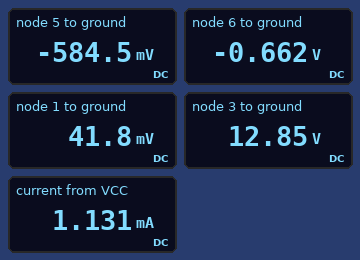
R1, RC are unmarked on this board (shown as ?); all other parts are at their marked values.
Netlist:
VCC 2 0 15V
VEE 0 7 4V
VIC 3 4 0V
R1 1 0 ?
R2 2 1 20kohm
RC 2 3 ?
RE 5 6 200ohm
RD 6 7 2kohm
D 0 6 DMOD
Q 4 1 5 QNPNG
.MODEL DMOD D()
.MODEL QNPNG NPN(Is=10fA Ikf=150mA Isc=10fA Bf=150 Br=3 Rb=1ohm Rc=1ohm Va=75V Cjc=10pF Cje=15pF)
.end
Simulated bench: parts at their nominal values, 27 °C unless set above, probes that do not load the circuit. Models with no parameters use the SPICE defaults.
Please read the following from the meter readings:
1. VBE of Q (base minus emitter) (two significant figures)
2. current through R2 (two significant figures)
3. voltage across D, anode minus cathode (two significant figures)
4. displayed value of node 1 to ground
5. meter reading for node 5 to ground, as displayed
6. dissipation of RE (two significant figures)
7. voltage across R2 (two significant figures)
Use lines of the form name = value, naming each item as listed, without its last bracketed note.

VBE of Q (base minus emitter) = 630 mV
current through R2 = 750 µA
voltage across D, anode minus cathode = 660 mV
displayed value of node 1 to ground = 41.8 mV
meter reading for node 5 to ground, as displayed = -584.5 mV
dissipation of RE = 30 µW
voltage across R2 = 15 V
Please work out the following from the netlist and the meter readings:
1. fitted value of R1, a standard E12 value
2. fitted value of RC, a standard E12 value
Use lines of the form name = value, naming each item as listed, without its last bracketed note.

fitted value of R1, a standard E12 value = 56 Ω
fitted value of RC, a standard E12 value = 5.6 kΩ
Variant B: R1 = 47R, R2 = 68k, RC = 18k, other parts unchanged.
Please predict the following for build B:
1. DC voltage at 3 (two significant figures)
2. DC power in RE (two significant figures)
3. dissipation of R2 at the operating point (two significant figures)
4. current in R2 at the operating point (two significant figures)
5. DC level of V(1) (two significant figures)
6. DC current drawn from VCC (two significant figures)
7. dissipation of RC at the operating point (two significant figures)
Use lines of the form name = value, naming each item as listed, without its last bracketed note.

DC voltage at 3 = 10 V
DC power in RE = 15 µW
dissipation of R2 at the operating point = 3.3 mW
current in R2 at the operating point = 220 µA
DC level of V(1) = 10 mV
DC current drawn from VCC = 500 µA
dissipation of RC at the operating point = 1.4 mW
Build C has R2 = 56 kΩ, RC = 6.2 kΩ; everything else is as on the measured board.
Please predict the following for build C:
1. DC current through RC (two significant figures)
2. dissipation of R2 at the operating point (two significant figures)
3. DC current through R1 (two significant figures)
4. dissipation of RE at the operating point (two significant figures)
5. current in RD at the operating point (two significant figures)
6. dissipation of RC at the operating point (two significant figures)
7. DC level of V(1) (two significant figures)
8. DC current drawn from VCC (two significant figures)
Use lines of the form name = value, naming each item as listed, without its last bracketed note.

DC current through RC = 290 µA
dissipation of R2 at the operating point = 4.0 mW
DC current through R1 = 270 µA
dissipation of RE at the operating point = 17 µW
current in RD at the operating point = 1.7 mA
dissipation of RC at the operating point = 530 µW
DC level of V(1) = 15 mV
DC current drawn from VCC = 560 µA
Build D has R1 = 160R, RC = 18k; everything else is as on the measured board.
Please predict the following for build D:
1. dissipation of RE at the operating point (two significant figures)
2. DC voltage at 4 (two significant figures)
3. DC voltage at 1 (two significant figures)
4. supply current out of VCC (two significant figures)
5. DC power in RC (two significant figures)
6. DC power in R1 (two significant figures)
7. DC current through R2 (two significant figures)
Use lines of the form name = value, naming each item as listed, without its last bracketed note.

dissipation of RE at the operating point = 86 µW
DC voltage at 4 = 3.3 V
DC voltage at 1 = 120 mV
supply current out of VCC = 1.4 mA
DC power in RC = 7.6 mW
DC power in R1 = 88 µW
DC current through R2 = 740 µA
